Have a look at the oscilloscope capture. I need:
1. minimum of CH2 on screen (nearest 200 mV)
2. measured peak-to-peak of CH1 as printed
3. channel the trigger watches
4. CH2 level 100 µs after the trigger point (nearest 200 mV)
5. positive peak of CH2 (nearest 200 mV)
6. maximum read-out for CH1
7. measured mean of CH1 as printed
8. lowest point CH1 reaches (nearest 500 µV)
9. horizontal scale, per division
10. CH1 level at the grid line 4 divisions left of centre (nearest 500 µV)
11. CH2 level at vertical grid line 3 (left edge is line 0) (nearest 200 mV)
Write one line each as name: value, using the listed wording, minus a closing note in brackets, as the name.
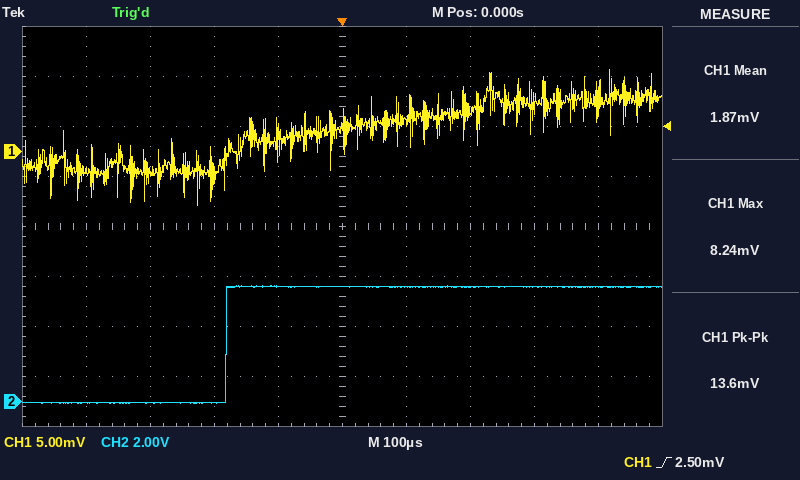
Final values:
minimum of CH2 on screen: 0.0 V
measured peak-to-peak of CH1 as printed: 13.6 mV
channel the trigger watches: CH1
CH2 level 100 µs after the trigger point: 4.6 V
positive peak of CH2: 4.6 V
maximum read-out for CH1: 8.24 mV
measured mean of CH1 as printed: 1.87 mV
lowest point CH1 reaches: -5.5 mV
horizontal scale, per division: 100 µs
CH1 level at the grid line 4 divisions left of centre: -2.0 mV
CH2 level at vertical grid line 3 (left edge is line 0): 0.0 V
